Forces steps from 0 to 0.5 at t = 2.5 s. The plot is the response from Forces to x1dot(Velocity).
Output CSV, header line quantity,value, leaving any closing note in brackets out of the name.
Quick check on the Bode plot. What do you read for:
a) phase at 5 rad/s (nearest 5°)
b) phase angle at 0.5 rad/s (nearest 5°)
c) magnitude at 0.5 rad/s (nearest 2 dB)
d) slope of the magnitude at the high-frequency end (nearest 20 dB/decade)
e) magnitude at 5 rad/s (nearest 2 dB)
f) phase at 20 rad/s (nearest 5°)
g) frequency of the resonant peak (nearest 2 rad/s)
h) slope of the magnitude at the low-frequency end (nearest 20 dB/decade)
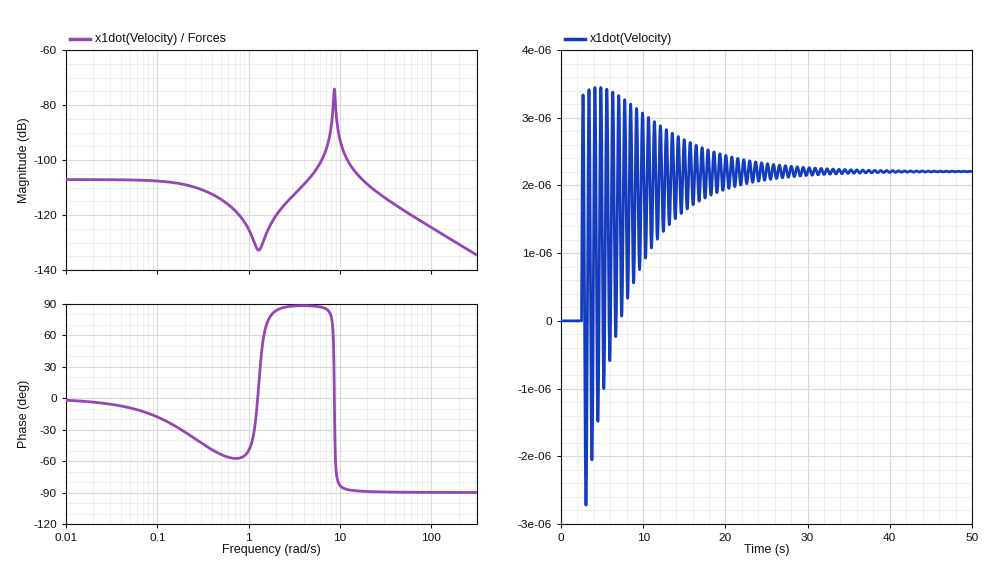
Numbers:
quantity,value
phase at 5 rad/s,90°
phase angle at 0.5 rad/s,-55°
magnitude at 0.5 rad/s,-114 dB
slope of the magnitude at the high-frequency end,-20 dB/decade
magnitude at 5 rad/s,-106 dB
phase at 20 rad/s,-90°
frequency of the resonant peak,8 rad/s
slope of the magnitude at the low-frequency end,0 dB/decade
